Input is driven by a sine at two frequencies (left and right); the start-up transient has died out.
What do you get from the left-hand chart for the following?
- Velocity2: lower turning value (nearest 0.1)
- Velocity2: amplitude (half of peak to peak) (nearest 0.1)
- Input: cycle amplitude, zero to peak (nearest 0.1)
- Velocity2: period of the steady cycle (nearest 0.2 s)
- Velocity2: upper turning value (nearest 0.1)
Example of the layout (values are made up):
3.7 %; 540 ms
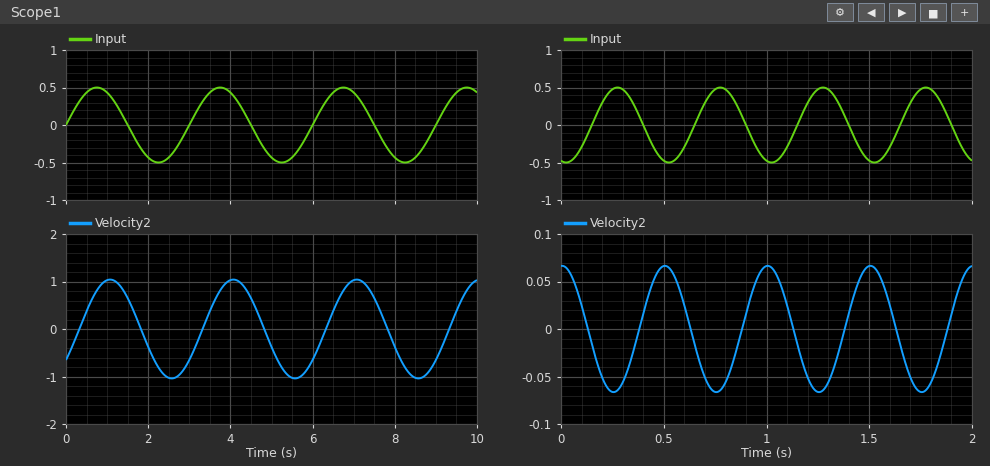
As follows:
-1.0; 1.0; 0.5; 3.0 s; 1.0
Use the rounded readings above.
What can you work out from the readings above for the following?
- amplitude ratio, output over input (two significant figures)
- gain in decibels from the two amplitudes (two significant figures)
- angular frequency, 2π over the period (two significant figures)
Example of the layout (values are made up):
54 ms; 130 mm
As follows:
2.0; 6.0 dB; 2.1 rad/s
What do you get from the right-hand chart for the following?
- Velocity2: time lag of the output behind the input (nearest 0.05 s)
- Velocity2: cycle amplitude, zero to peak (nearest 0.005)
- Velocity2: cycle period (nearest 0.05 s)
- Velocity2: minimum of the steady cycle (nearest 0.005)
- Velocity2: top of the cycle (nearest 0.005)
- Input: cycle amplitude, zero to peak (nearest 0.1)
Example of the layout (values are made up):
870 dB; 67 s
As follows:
0.25 s; 0.065; 0.50 s; -0.065; 0.065; 0.5
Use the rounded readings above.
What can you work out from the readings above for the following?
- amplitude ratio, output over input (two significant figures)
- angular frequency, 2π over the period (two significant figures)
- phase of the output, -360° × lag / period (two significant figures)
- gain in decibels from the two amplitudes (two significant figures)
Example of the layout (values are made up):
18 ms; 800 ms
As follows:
0.13; 13 rad/s; -180°; -18 dB
